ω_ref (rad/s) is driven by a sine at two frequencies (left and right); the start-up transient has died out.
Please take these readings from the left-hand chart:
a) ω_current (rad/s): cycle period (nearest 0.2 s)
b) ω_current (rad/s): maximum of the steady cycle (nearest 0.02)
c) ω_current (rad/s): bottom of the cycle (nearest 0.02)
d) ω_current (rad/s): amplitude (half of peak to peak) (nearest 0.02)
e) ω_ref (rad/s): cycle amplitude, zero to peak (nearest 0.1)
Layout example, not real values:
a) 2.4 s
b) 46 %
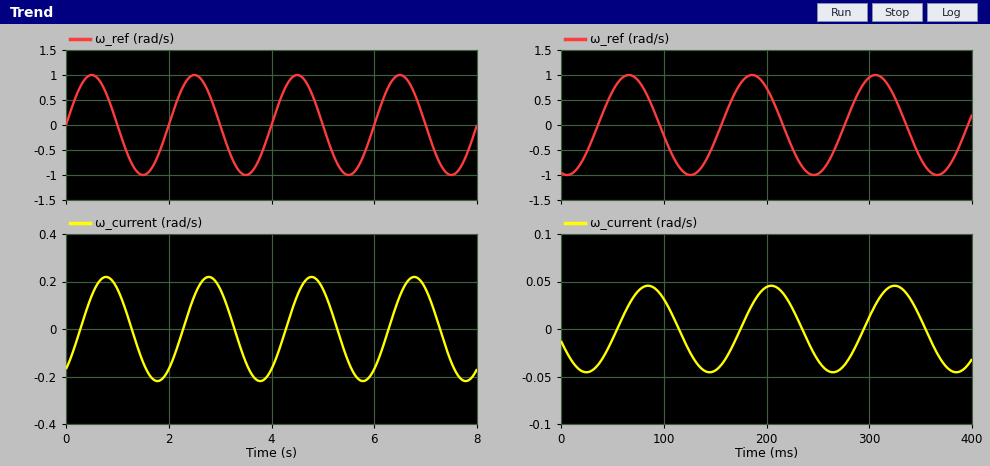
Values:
a) 2.0 s
b) 0.22
c) -0.22
d) 0.22
e) 1.0
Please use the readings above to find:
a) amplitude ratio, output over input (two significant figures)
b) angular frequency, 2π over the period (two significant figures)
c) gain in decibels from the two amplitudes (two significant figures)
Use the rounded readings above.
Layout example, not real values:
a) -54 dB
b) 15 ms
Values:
a) 0.22
b) 3.1 rad/s
c) -13 dB
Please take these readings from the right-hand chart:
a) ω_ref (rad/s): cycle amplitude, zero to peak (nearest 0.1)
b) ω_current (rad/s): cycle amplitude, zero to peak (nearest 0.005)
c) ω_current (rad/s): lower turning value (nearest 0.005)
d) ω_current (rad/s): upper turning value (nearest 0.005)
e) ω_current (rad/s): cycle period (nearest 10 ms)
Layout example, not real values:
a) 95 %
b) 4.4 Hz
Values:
a) 1.0
b) 0.045
c) -0.045
d) 0.045
e) 120 ms
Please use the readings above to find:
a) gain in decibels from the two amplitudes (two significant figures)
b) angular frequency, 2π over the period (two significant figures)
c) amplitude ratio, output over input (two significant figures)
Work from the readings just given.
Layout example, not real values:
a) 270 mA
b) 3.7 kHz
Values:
a) -27 dB
b) 0.052 rad/ms
c) 0.045
